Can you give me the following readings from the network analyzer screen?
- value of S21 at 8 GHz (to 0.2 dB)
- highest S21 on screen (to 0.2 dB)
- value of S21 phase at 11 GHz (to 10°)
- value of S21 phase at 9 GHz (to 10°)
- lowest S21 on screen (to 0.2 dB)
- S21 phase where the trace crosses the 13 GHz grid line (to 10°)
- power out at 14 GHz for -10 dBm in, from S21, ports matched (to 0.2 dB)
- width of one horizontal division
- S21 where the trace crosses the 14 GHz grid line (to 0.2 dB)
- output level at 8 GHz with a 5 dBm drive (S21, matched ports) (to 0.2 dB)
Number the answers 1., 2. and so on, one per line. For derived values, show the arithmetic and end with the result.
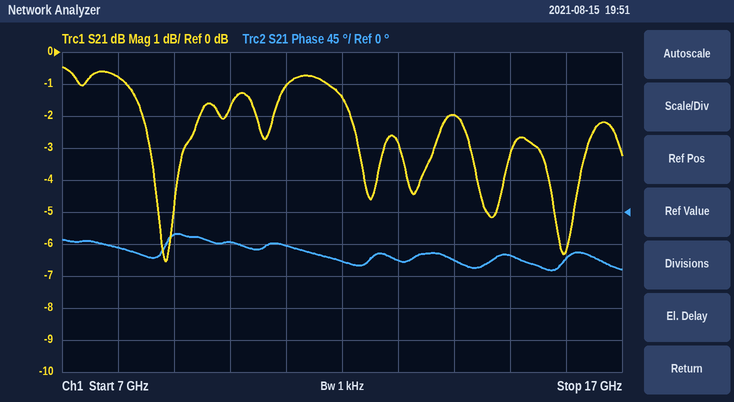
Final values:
1. -0.8 dB
2. -0.4 dB
3. -50°
4. -30°
5. -6.6 dB
6. -70°
7. -10 dBm + (-2.0 dB) = -12.0 dBm
8. 1 GHz
9. -2.0 dB
10. 5 dBm + (-0.8 dB) = 4.2 dBm
